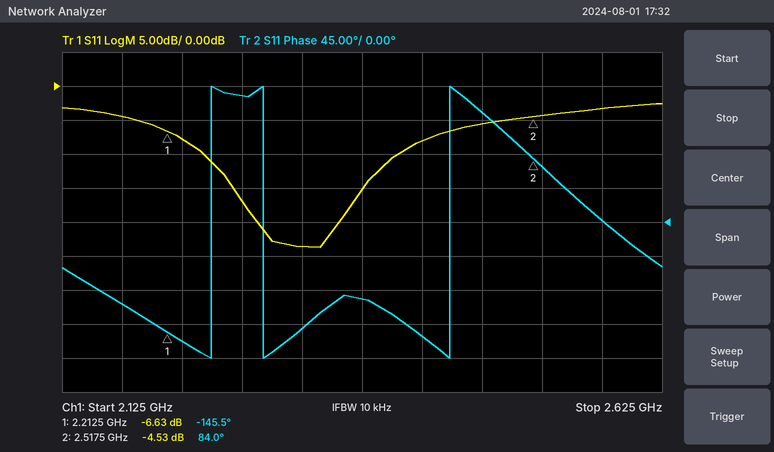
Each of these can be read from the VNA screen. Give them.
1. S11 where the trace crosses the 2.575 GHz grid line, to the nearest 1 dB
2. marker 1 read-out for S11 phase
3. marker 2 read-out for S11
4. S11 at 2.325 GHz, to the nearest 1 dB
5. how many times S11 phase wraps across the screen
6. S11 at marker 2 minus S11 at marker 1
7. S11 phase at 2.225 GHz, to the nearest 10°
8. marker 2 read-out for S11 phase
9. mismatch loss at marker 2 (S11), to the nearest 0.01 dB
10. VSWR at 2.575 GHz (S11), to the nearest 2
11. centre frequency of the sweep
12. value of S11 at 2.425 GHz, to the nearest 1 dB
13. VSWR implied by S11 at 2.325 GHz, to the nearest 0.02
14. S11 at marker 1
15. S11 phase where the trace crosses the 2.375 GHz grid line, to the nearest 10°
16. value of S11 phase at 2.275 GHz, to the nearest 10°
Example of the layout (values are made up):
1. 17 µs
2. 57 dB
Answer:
1. -3 dB
2. -145.5°
3. -4.53 dB
4. -24 dB
5. 3
6. 2.10 dB
7. -160°
8. 84.0°
9. 1.89 dB
10. 6
11. 2.375 GHz
12. -8 dB
13. 1.14
14. -6.63 dB
15. -100°
16. 170°
